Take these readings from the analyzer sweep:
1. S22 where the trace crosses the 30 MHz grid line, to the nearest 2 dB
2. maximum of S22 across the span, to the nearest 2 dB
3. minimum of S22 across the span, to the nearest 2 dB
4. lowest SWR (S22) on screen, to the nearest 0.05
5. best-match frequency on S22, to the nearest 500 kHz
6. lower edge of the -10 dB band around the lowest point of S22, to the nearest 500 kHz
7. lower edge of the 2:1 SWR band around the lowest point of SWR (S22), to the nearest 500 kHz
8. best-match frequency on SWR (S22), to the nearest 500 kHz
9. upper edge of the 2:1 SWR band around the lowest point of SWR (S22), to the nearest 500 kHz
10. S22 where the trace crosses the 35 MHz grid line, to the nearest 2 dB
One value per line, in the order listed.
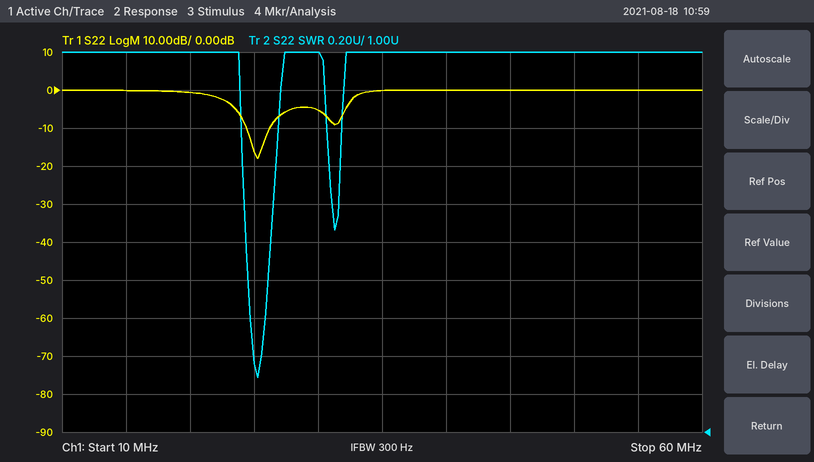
-6 dB
0 dB
-18 dB
1.30
25.5 MHz
24.5 MHz
24.5 MHz
25.5 MHz
26.5 MHz
0 dB
